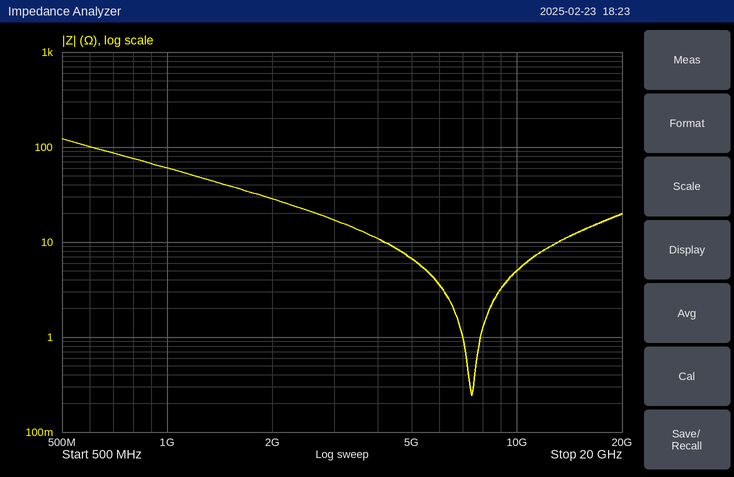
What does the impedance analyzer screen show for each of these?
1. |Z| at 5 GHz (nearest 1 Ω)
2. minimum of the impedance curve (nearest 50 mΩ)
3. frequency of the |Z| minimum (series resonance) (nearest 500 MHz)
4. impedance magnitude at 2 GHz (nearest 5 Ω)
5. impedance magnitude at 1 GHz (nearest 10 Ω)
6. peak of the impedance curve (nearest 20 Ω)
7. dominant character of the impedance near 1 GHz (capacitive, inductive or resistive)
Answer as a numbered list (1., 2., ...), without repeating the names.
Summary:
1. 7 Ω
2. 250 mΩ
3. 7.5 GHz
4. 30 Ω
5. 60 Ω
6. 120 Ω
7. capacitive
